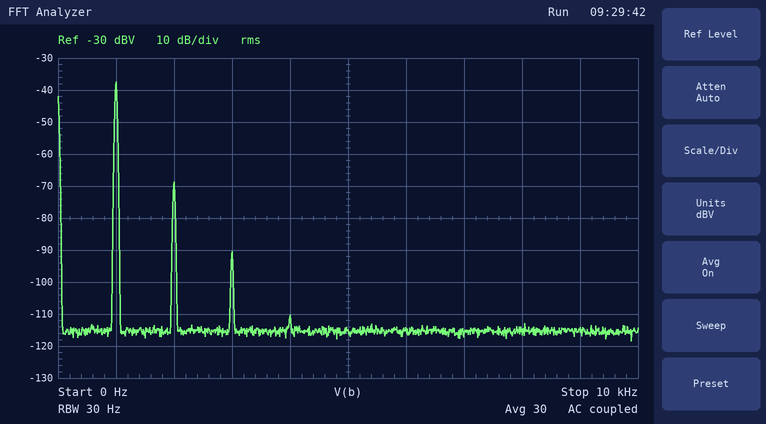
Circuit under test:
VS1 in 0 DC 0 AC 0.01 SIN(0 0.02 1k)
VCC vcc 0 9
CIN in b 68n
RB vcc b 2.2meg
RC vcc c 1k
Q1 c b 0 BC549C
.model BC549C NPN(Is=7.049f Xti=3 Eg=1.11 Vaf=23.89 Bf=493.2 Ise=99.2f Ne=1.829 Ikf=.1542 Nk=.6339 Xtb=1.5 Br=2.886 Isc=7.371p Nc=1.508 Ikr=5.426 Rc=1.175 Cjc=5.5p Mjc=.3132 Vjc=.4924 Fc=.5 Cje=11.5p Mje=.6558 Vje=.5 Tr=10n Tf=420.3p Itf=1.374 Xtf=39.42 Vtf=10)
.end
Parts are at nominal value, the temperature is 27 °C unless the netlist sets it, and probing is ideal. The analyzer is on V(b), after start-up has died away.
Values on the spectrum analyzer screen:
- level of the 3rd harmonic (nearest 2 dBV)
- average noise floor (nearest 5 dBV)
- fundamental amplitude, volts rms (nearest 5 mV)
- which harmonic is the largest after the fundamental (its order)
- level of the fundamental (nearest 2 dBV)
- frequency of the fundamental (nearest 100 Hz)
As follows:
-90 dBV
-115 dBV
15 mV
2
-38 dBV
1.0 kHz
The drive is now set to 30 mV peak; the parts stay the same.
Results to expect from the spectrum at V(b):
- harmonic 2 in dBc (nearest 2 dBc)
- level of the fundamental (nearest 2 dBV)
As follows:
-28 dBc
-34 dBV
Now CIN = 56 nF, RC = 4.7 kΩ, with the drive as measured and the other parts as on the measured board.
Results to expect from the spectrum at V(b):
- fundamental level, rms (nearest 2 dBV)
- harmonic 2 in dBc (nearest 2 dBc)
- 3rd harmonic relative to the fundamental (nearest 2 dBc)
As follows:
-40 dBV
-16 dBc
-24 dBc
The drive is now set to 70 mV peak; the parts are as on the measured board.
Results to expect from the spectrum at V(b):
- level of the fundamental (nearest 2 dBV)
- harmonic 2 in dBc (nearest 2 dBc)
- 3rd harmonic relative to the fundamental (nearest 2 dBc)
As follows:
-26 dBV
-26 dBc
-38 dBc
